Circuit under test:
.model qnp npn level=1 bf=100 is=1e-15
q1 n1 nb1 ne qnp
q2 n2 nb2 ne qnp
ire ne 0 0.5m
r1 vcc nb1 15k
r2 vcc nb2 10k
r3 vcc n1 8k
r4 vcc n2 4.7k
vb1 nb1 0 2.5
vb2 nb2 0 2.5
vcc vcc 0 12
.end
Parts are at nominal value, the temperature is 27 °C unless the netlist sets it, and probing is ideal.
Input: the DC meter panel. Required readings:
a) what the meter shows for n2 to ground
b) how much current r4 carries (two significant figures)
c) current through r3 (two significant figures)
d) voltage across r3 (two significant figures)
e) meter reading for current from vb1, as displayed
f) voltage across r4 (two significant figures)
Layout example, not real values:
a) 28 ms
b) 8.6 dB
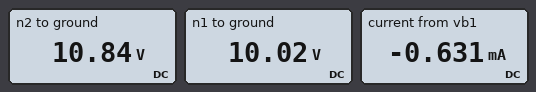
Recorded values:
a) 10.84 V
b) 250 µA
c) 250 µA
d) 2.0 V
e) -0.631 mA
f) 1.2 V
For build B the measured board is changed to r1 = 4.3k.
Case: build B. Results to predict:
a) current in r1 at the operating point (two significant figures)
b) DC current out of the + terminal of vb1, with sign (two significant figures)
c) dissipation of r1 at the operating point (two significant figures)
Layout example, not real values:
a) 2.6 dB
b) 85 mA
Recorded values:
a) 2.2 mA
b) -2.2 mA
c) 21 mW
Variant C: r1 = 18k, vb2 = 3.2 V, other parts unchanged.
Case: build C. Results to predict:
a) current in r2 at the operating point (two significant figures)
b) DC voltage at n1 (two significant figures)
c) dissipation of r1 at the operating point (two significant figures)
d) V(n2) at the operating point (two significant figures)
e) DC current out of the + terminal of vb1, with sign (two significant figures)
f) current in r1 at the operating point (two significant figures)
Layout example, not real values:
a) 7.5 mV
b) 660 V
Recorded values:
a) 880 µA
b) 12 V
c) 5.0 mW
d) 9.7 V
e) -530 µA
f) 530 µA
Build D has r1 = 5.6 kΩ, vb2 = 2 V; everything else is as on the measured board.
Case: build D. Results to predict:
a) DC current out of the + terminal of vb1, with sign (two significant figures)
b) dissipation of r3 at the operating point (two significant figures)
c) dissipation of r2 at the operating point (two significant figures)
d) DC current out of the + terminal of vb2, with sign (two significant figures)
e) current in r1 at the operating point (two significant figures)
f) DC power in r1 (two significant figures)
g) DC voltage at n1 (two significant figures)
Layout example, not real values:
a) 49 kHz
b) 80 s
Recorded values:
a) -1.7 mA
b) 2.0 mW
c) 10 mW
d) -1.0 mA
e) 1.7 mA
f) 16 mW
g) 8.0 V
